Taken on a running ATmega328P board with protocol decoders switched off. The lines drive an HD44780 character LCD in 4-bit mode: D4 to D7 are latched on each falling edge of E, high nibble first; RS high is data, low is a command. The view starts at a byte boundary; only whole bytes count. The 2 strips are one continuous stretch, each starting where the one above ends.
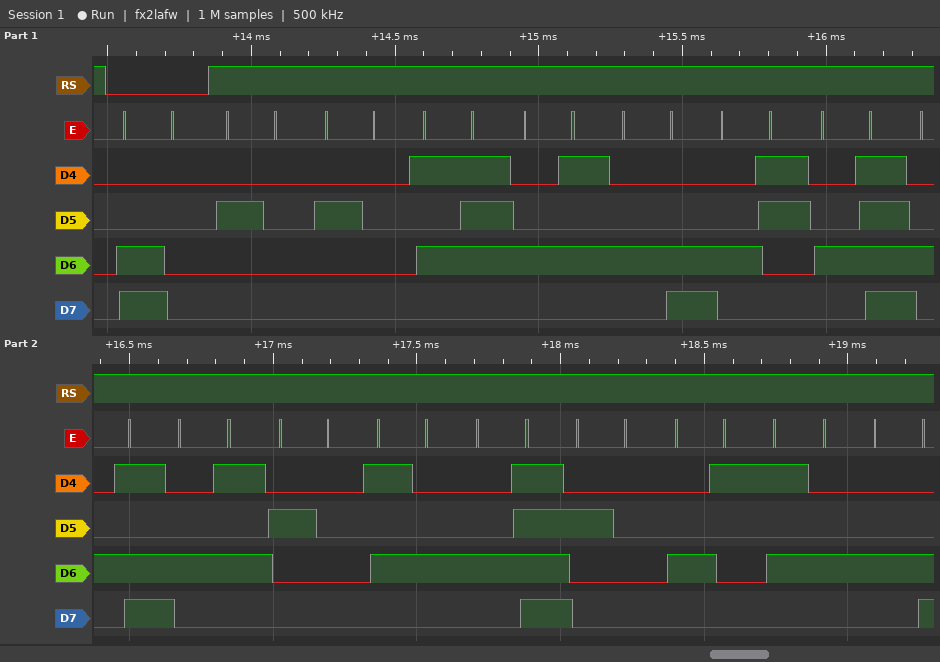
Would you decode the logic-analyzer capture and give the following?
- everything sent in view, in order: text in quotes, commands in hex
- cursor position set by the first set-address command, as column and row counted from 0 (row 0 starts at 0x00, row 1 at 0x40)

0xC0 "  WELCOME TO ATL"
column 0, row 1
